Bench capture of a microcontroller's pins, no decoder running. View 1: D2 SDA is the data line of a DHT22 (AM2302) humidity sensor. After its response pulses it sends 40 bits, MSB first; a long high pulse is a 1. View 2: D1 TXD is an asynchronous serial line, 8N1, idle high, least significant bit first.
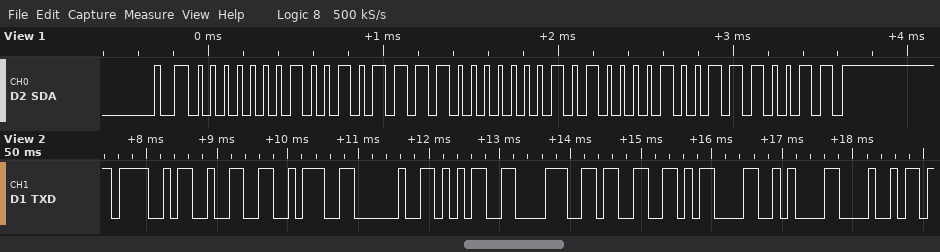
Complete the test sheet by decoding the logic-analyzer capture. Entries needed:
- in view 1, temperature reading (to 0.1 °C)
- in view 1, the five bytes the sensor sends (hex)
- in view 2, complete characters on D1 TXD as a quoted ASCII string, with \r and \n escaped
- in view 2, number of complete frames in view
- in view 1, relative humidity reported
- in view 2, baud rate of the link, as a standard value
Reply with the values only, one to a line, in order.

32.2 °C
01 2F 01 42 73
"O2: 583\r\nH"
10
30.3 %
9600 baud
